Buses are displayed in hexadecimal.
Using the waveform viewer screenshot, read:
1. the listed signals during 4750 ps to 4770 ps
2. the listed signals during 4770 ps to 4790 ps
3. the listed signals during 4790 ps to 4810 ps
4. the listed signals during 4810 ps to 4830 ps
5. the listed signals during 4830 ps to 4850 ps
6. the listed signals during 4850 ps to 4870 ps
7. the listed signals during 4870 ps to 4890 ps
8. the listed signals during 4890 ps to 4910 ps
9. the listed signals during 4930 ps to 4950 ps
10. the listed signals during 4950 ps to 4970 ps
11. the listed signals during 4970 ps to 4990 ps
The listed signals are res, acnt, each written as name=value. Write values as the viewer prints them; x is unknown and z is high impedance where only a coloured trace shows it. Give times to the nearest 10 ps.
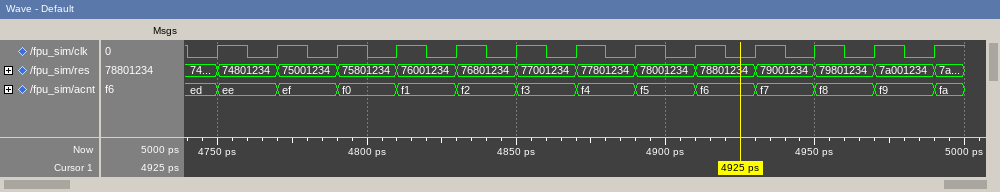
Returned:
res=74801234, acnt=ee
res=75001234, acnt=ef
res=75801234, acnt=f0
res=76001234, acnt=f1
res=76801234, acnt=f2
res=77001234, acnt=f3
res=77801234, acnt=f4
res=78001234, acnt=f5
res=79001234, acnt=f7
res=79801234, acnt=f8
res=7a001234, acnt=f9
